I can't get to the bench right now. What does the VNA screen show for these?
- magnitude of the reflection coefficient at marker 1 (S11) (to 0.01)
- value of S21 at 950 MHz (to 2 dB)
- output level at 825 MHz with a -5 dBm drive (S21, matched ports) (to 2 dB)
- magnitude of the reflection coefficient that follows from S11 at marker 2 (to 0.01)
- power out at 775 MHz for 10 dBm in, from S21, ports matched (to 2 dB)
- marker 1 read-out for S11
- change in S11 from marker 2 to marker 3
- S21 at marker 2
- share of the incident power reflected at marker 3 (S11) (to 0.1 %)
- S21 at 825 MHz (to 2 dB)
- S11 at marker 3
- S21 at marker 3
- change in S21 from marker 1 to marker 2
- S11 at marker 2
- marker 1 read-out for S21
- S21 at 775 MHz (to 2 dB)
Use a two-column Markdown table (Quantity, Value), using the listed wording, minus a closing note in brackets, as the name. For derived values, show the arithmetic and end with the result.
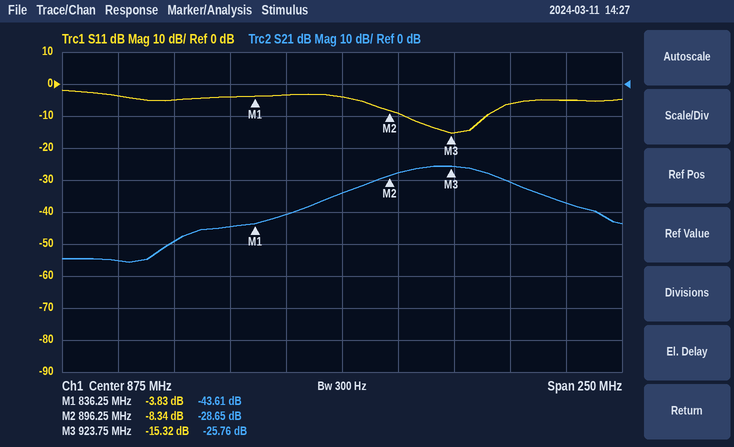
| Quantity | Value |
|---|---|
| magnitude of the reflection coefficient at marker 1 (S11) | 10^(-3.83/20) ≈ 0.64 |
| value of S21 at 950 MHz | -30 dB |
| output level at 825 MHz with a -5 dBm drive (S21, matched ports) | -5 dBm + (-44 dB) = -50 dBm |
| magnitude of the reflection coefficient that follows from S11 at marker 2 | 10^(-8.34/20) ≈ 0.38 |
| power out at 775 MHz for 10 dBm in, from S21, ports matched | 10 dBm + (-56 dB) = -46 dBm |
| marker 1 read-out for S11 | -3.83 dB |
| change in S11 from marker 2 to marker 3 | -15.32 − (-8.34) = -6.98 dB |
| S21 at marker 2 | -28.65 dB |
| share of the incident power reflected at marker 3 (S11) | 10^(-15.32/10) ≈ 2.9 % |
| S21 at 825 MHz | -44 dB |
| S11 at marker 3 | -15.32 dB |
| S21 at marker 3 | -25.76 dB |
| change in S21 from marker 1 to marker 2 | -28.65 − (-43.61) = 14.96 dB |
| S11 at marker 2 | -8.34 dB |
| marker 1 read-out for S21 | -43.61 dB |
| S21 at 775 MHz | -56 dB |
